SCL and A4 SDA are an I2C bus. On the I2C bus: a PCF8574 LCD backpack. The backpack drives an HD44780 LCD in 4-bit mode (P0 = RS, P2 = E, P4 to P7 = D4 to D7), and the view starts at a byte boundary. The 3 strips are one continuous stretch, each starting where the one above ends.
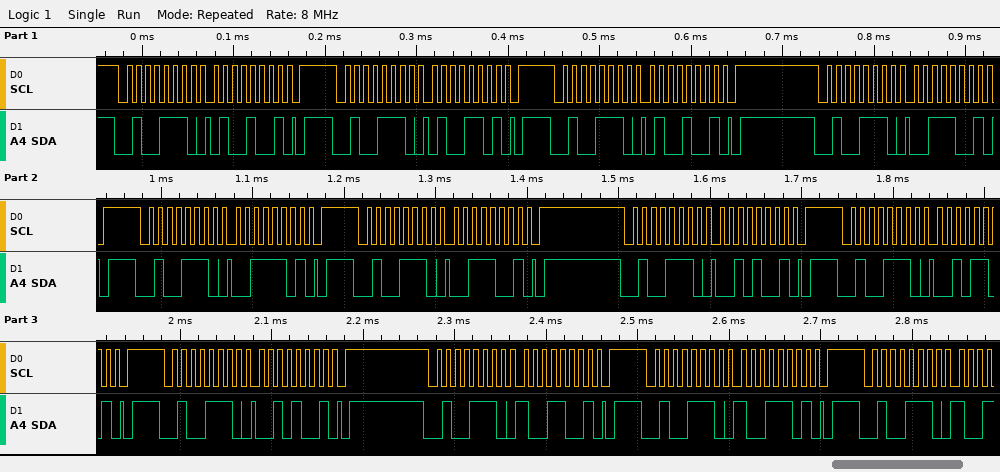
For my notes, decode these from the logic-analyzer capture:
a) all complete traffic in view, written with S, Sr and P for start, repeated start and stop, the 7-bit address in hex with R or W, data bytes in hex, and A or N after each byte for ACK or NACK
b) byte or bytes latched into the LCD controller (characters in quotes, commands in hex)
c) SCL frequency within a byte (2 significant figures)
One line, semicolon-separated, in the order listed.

S 27W A 49 A P S 27W A 4D A P S 27W A 49 A P S 27W A 39 A P S 27W A 3D A P S 27W A 39 A P S 27W A 29 A P S 27W A 2D A P S 27W A 29 A P S 27W A 99 A P S 27W A 9D A P S 27W A; 'C'; 100 kHz
